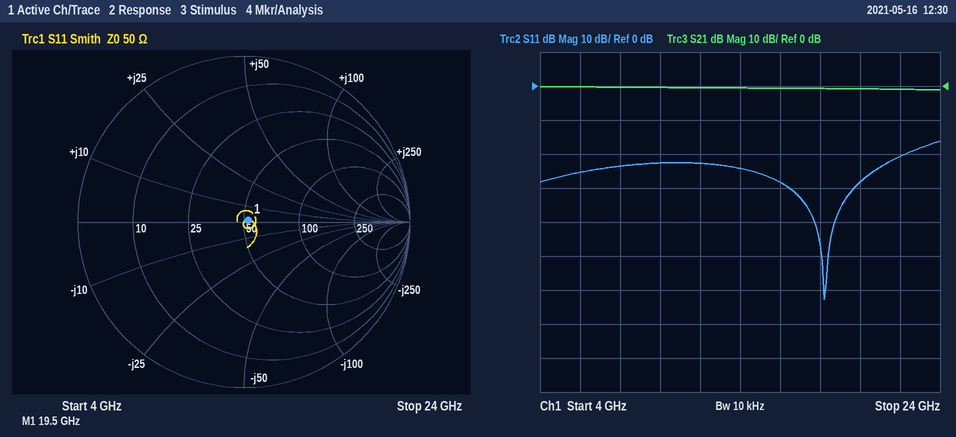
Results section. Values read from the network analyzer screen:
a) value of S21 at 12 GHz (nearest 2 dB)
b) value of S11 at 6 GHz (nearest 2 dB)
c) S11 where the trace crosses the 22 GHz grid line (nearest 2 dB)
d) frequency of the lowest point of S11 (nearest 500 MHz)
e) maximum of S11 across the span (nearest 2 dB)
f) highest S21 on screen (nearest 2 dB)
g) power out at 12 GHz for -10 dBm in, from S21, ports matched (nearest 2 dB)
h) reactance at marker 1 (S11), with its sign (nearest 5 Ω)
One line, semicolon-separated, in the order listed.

0 dB; -26 dB; -20 dB; 18.0 GHz; -16 dB; 0 dB; -10 dBm; 0 Ω
